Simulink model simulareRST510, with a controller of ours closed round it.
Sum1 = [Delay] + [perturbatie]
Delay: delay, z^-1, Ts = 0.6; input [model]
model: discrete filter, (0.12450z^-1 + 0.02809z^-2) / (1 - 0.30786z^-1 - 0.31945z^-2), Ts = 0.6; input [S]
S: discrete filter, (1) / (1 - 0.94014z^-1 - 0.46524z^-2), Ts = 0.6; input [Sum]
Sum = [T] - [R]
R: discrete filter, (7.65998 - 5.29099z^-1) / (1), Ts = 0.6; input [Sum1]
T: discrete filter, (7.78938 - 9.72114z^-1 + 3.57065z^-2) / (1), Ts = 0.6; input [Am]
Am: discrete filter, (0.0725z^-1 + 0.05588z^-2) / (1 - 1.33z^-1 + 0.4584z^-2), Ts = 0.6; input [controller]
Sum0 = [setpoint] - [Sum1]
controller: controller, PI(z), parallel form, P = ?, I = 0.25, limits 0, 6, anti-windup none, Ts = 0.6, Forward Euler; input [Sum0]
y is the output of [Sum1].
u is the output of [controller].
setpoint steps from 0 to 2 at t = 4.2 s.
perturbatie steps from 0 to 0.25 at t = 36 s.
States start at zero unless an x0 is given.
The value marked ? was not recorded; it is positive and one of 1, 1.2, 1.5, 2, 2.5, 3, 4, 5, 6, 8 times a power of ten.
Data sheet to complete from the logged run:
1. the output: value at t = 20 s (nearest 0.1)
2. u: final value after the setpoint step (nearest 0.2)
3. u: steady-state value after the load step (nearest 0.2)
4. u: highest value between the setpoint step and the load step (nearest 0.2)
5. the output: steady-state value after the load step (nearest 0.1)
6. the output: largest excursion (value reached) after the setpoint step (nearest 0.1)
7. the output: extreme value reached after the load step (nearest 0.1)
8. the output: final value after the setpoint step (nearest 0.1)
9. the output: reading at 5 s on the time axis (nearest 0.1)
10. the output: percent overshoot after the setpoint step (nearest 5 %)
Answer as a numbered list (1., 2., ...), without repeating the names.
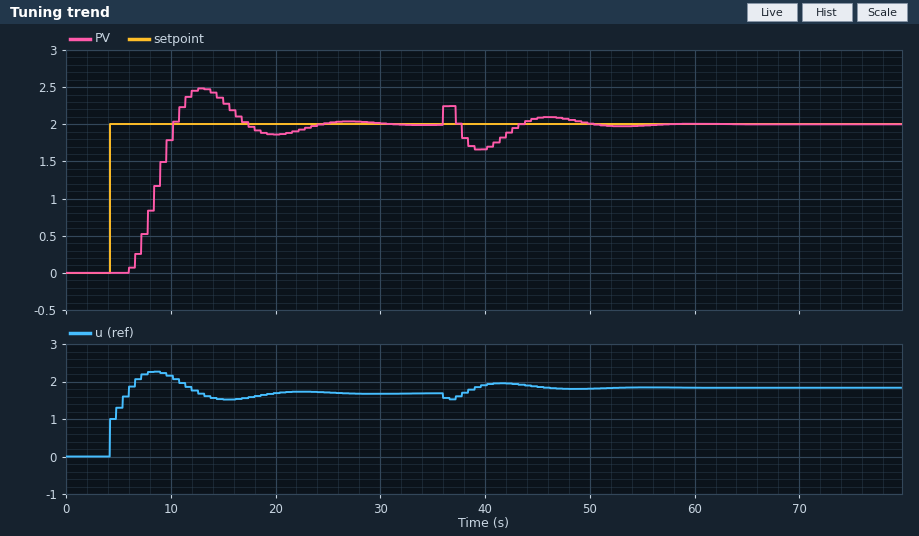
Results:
1. 1.9
2. 1.6
3. 1.8
4. 2.2
5. 2.0
6. 2.5
7. 1.7
8. 2.0
9. 0.0
10. 25 %
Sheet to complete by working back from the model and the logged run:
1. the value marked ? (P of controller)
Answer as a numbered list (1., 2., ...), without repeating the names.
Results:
1. 0.5
